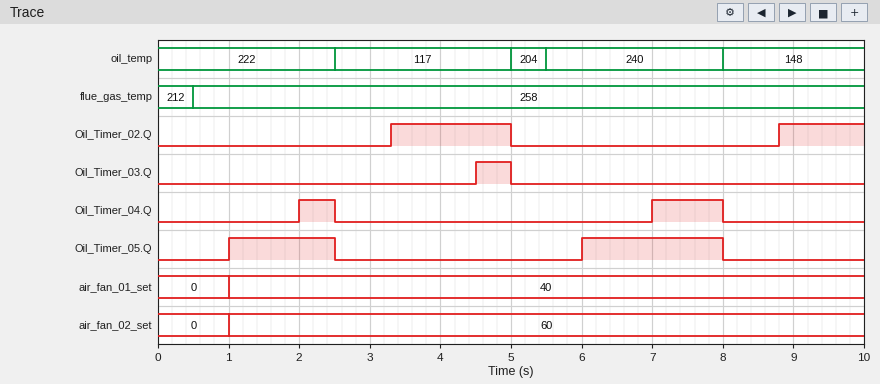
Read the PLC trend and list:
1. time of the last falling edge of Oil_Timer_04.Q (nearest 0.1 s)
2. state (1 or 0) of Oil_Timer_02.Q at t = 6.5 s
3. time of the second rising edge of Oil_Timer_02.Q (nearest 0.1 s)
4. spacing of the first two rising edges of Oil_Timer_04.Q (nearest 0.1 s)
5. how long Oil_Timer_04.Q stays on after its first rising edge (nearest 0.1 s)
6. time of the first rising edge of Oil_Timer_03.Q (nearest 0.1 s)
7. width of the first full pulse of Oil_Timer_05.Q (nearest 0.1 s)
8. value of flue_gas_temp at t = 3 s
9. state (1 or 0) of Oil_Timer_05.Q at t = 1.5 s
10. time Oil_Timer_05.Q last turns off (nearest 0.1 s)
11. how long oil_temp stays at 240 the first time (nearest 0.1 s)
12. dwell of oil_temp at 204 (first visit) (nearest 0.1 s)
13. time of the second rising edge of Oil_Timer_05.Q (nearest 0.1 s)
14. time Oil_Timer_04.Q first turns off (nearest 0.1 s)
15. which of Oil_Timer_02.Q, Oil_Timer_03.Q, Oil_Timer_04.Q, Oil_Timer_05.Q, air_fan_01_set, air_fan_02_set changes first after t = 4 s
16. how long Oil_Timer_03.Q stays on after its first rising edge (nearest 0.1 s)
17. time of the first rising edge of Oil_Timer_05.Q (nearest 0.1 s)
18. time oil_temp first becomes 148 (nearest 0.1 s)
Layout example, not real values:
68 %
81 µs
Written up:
8.0 s
0
8.8 s
5.0 s
0.5 s
4.5 s
1.5 s
258
1
8.0 s
2.5 s
0.5 s
6.0 s
2.5 s
Oil_Timer_03.Q
0.5 s
1.0 s
8.0 s
